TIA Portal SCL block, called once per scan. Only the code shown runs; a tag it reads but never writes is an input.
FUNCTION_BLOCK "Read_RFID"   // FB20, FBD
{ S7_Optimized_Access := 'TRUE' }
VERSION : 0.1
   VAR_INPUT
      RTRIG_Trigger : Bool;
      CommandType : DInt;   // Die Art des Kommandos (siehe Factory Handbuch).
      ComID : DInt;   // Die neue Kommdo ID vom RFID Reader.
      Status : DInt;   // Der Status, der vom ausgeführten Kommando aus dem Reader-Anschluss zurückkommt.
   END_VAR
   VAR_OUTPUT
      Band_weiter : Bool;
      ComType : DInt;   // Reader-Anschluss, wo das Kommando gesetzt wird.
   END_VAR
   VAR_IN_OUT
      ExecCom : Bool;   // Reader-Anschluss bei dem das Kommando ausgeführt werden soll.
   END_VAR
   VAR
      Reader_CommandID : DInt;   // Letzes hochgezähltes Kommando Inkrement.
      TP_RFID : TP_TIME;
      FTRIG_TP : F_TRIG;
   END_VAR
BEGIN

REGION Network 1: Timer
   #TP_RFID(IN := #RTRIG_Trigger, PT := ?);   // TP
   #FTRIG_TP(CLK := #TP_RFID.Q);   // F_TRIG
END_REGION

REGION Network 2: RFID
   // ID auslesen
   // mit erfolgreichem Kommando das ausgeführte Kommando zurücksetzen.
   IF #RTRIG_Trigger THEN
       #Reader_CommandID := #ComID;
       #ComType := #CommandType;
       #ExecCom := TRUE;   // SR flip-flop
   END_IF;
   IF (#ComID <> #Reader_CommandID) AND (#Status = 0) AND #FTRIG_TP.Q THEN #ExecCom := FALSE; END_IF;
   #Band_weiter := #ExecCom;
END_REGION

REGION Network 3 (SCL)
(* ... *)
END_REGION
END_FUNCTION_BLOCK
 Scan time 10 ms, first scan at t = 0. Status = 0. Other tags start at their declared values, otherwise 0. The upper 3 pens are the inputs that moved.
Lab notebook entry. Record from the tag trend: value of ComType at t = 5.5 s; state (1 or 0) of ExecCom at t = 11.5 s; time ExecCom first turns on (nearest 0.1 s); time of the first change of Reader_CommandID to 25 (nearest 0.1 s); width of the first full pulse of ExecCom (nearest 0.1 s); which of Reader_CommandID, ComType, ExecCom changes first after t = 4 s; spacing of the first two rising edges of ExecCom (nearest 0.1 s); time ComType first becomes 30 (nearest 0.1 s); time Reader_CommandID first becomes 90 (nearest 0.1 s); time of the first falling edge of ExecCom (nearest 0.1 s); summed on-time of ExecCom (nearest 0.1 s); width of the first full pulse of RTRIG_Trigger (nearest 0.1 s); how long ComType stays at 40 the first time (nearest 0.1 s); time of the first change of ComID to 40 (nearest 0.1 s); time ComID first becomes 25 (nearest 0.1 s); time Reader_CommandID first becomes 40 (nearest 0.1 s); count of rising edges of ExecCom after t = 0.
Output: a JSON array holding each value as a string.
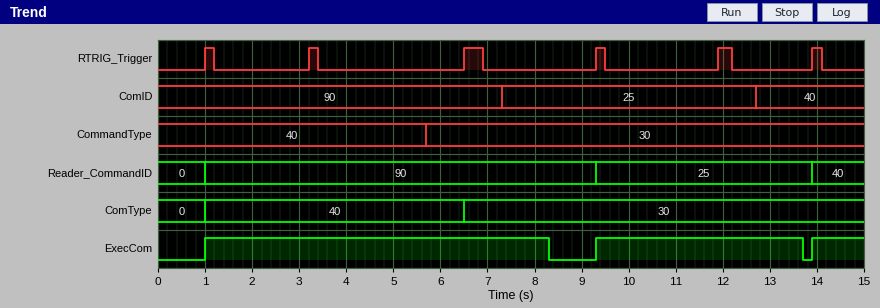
["40", "1", "1.0 s", "9.3 s", "7.3 s", "ComType", "8.3 s", "6.5 s", "1.0 s", "8.3 s", "12.8 s", "0.2 s", "5.5 s", "12.7 s", "7.3 s", "13.9 s", "3"]
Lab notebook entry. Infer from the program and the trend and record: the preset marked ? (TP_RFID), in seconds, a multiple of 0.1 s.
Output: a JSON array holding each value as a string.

["1.8 s"]
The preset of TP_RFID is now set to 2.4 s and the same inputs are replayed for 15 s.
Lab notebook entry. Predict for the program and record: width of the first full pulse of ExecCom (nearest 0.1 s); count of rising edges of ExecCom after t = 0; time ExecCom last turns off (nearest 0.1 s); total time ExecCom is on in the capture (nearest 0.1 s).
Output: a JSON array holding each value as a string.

["7.9 s", "2", "8.9 s", "13.6 s"]
